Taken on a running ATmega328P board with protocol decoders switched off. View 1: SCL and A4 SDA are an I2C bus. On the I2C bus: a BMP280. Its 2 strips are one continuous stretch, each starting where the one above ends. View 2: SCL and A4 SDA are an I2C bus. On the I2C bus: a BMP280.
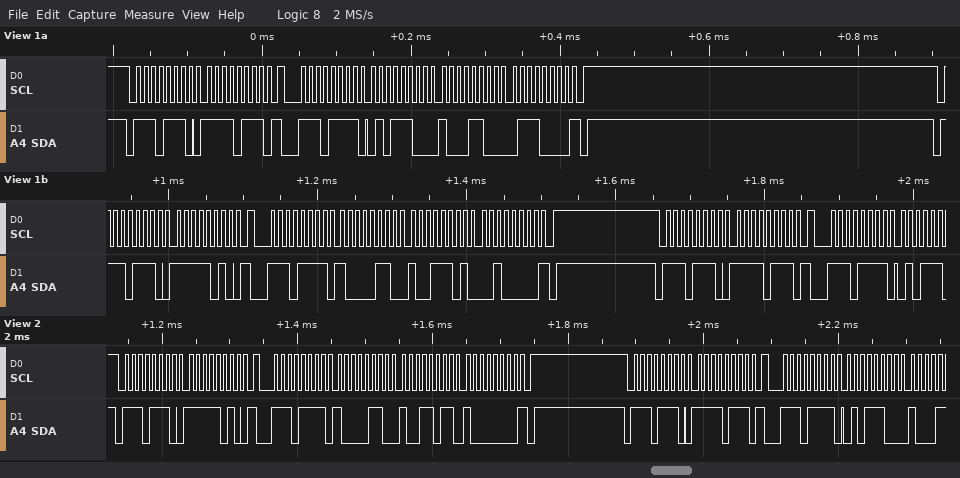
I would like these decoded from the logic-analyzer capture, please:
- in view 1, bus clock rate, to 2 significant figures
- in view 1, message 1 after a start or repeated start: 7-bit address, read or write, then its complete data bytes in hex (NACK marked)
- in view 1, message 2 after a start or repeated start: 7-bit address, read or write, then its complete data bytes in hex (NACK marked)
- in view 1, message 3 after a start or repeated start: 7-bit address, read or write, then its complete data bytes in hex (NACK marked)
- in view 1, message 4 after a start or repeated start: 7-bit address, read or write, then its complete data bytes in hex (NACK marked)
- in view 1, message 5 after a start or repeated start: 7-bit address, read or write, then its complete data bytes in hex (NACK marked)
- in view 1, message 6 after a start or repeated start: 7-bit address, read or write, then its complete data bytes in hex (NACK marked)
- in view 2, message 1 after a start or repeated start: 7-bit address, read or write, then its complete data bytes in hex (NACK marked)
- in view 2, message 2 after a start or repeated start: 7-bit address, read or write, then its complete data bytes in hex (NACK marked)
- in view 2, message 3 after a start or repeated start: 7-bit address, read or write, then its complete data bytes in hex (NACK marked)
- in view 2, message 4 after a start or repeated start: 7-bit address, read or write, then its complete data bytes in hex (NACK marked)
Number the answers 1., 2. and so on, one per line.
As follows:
1. 100 kHz
2. 0x77 write: F7
3. 0x77 read: 5C 8C 70 NACK
4. 0x77 write: FA
5. 0x77 read: 86 9D 20 NACK
6. 0x77 write: F7
7. 0x77 read
8. 0x77 write: FA
9. 0x77 read: 86 9B 80 NACK
10. 0x77 write: F7
11. 0x77 read: 5C
